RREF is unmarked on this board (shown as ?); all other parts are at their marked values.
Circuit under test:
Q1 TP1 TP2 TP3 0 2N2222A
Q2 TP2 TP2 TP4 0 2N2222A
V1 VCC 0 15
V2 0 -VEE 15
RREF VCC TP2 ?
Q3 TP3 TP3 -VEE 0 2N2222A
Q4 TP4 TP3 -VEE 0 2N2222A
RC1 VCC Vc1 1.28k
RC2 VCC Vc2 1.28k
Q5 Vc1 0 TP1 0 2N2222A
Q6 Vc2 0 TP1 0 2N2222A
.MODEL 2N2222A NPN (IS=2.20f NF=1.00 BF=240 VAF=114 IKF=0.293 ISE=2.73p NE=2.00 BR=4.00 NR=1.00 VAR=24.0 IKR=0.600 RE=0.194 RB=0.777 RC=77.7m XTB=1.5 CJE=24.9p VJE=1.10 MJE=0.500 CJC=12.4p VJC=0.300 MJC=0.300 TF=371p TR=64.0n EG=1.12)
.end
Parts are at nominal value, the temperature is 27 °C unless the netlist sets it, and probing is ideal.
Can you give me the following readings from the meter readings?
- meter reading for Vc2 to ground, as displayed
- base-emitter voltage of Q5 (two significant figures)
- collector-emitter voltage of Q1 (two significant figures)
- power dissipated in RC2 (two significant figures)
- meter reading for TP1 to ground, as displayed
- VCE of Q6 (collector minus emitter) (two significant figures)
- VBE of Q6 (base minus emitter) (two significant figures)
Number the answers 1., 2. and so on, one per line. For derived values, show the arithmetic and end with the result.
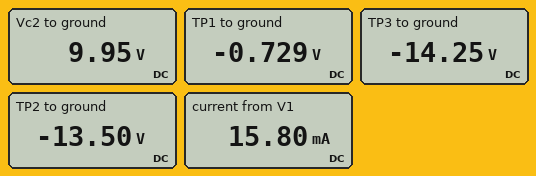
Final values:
1. 9.95 V
2. 0 V - (-729 mV) = 730 mV
3. -729 mV - (-14.25 V) = 14 V
4. (15 V - 9.95 V)^2 / 1.28 kΩ = 20 mW
5. -0.729 V
6. 9.95 V - (-729 mV) = 11 V
7. 0 V - (-729 mV) = 730 mV
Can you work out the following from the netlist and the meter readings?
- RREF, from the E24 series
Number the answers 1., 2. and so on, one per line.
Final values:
1. 3.6 kΩ
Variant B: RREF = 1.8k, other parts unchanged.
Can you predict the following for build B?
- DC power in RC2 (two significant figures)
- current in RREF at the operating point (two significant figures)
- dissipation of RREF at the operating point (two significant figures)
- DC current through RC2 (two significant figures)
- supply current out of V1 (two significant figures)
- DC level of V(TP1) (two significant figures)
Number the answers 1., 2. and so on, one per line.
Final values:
1. 79 mW
2. 16 mA
3. 450 mW
4. 7.9 mA
5. 32 mA
6. -750 mV
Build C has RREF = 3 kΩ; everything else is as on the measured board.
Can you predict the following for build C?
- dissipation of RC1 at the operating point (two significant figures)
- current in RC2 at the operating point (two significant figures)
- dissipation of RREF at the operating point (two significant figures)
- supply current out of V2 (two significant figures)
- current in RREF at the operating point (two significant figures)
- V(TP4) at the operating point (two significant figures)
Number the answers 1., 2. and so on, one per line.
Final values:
1. 29 mW
2. 4.7 mA
3. 270 mW
4. 19 mA
5. 9.5 mA
6. -14 V
